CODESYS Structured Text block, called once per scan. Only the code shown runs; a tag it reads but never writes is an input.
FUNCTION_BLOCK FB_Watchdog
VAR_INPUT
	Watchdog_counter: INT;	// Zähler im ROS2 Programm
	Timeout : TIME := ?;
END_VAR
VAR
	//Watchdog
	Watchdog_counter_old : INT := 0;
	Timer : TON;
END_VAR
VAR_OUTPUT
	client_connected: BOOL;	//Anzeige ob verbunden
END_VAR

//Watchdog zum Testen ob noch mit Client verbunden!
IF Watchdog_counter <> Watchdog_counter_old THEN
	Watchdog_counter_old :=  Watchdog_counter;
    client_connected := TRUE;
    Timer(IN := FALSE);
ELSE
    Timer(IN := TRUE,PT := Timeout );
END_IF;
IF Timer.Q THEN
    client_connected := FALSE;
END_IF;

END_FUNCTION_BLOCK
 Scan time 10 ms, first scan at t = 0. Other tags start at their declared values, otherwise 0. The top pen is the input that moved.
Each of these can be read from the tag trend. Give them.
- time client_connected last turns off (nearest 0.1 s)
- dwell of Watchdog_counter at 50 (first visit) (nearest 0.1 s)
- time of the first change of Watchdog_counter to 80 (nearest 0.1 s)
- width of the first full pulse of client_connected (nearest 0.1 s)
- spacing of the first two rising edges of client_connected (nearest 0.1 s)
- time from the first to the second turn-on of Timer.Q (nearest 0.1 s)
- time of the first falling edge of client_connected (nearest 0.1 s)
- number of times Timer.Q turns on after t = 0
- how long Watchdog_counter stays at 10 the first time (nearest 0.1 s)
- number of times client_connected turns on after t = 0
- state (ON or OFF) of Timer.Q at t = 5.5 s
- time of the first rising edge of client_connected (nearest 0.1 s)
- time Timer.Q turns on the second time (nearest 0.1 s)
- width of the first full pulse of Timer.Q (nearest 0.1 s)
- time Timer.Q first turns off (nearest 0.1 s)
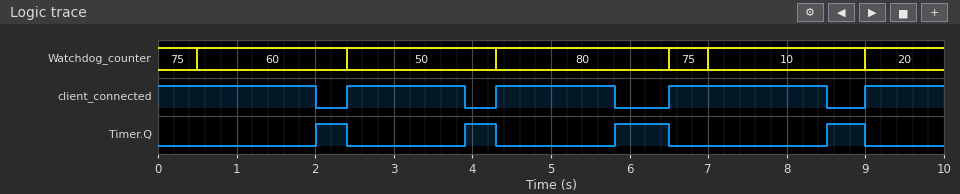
8.5 s
1.9 s
4.3 s
1.5 s
1.9 s
1.9 s
2.0 s
4
2.0 s
4
OFF
2.4 s
3.9 s
0.4 s
2.4 s
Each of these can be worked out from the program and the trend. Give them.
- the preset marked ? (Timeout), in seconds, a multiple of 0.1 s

1.5 s
